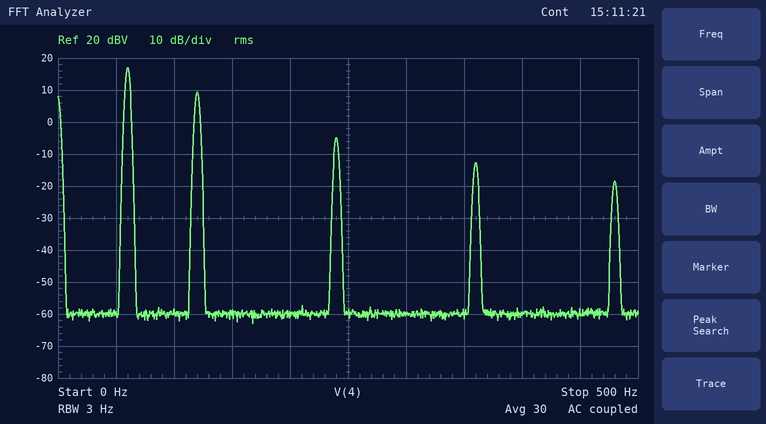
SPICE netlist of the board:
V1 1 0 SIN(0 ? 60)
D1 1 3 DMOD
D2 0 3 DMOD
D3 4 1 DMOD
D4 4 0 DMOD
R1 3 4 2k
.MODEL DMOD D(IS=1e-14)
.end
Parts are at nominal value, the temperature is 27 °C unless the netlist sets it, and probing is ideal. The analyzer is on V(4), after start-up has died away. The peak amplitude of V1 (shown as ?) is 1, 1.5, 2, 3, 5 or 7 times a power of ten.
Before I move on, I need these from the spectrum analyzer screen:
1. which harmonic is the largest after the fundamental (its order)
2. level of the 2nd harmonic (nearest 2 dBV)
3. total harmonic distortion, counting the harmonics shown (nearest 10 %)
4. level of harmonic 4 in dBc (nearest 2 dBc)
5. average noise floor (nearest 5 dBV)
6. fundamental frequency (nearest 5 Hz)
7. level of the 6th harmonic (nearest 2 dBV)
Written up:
2
10 dBV
40 %
-22 dBc
-60 dBV
60 Hz
-12 dBV
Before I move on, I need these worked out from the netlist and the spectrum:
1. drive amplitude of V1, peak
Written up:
20 V
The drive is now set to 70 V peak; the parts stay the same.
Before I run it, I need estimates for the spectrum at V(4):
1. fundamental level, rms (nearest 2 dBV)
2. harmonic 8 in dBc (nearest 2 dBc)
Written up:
28 dBV
-34 dBc
